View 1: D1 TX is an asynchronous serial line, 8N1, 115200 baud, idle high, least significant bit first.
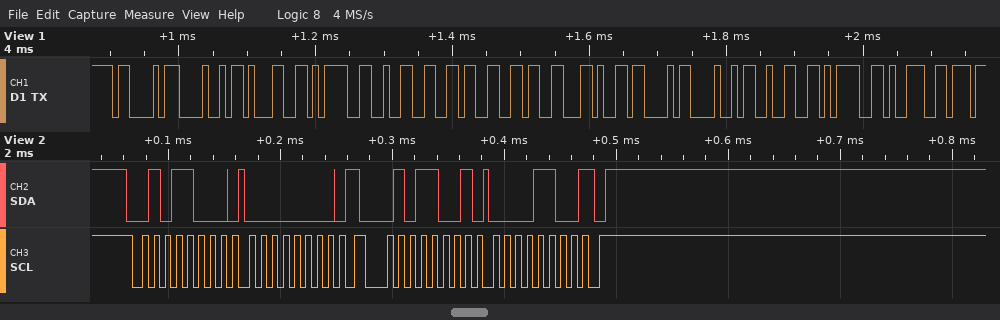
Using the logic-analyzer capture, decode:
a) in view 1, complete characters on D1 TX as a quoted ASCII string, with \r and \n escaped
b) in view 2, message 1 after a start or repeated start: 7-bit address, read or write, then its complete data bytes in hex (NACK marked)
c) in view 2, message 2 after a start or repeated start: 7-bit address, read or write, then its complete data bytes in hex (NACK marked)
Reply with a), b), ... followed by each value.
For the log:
a) "CH1=266,CH2=9"
b) 0x2C write: 00
c) 0x2C read: 0C NACK
